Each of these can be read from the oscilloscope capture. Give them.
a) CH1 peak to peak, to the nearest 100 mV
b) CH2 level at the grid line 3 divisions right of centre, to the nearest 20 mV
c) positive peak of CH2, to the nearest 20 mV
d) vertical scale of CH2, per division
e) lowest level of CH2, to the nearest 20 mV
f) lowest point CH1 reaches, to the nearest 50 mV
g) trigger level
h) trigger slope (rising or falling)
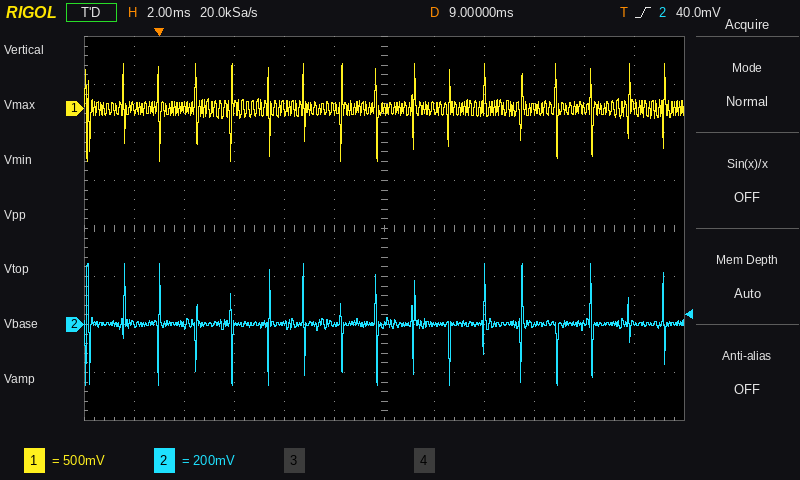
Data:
1.00 V
0 mV
260 mV
200 mV
-260 mV
-550 mV
40.0 mV
rising
